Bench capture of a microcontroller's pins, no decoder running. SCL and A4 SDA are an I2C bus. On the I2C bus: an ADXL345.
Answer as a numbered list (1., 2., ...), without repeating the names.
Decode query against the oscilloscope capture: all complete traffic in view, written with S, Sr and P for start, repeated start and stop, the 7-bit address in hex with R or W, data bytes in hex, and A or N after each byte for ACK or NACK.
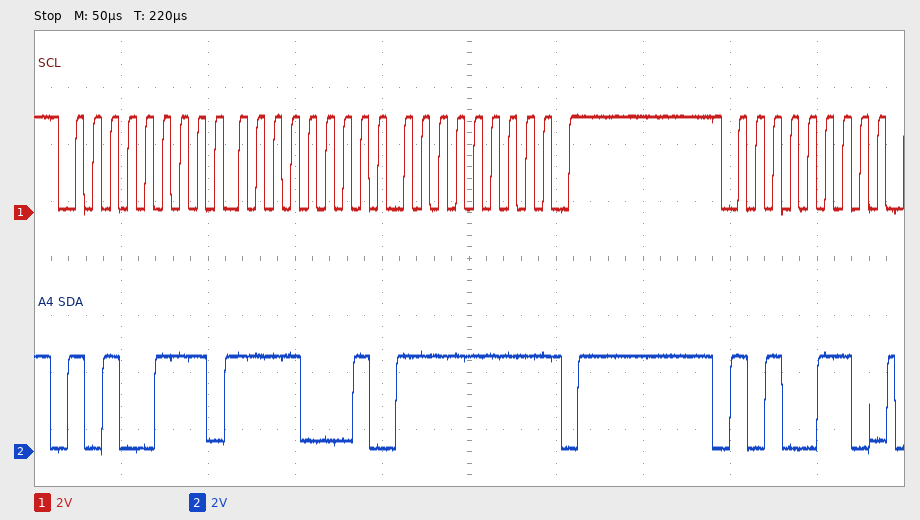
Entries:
1. S 53R A F1 A FF N P S 53W A
